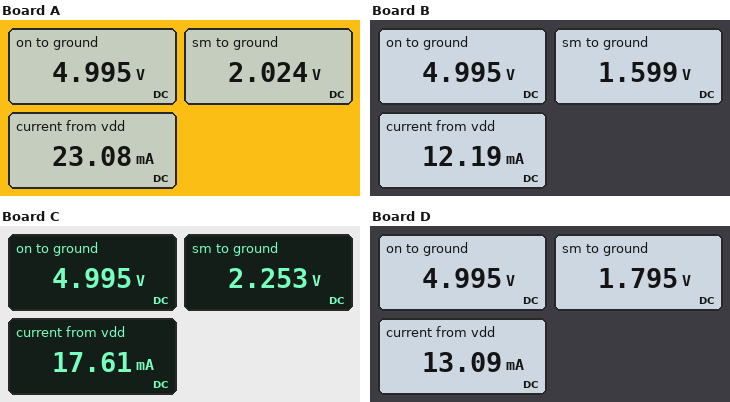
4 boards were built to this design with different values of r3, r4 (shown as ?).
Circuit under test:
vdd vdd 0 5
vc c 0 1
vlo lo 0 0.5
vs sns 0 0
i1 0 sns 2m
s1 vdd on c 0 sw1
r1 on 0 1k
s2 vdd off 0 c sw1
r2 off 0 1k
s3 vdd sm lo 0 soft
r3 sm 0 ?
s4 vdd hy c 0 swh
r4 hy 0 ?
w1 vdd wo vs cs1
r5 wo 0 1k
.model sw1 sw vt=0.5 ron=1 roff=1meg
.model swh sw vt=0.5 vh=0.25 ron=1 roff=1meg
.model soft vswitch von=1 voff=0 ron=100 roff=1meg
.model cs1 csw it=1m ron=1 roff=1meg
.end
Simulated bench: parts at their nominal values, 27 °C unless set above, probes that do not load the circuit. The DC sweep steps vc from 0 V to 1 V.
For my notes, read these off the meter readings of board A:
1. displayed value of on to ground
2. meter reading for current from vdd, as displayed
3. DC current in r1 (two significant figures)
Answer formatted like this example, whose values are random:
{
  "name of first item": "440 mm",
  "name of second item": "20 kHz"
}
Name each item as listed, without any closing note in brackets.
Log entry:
{
  "displayed value of on to ground": "4.995 V",
  "meter reading for current from vdd, as displayed": "23.08 mA",
  "DC current in r1": "5.0 mA"
}
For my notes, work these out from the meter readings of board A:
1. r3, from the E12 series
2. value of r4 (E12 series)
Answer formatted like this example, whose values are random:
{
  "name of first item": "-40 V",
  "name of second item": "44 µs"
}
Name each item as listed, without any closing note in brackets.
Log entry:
{
  "r3, from the E12 series": "6.8 kΩ",
  "value of r4": "390 Ω"
}
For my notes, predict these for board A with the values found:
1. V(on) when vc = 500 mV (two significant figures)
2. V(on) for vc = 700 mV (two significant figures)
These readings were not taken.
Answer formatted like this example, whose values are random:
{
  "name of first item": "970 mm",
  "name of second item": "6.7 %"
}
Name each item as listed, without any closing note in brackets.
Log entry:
{
  "V(on) when vc = 500 mV": "5.0 V",
  "V(on) for vc = 700 mV": "5.0 V"
}
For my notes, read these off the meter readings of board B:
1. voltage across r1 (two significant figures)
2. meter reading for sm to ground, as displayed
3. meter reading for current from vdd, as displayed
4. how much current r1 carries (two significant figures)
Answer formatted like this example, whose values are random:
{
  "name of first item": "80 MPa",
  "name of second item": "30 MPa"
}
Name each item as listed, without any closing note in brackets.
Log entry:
{
  "voltage across r1": "5.0 V",
  "meter reading for sm to ground, as displayed": "1.599 V",
  "meter reading for current from vdd, as displayed": "12.19 mA",
  "how much current r1 carries": "5.0 mA"
}
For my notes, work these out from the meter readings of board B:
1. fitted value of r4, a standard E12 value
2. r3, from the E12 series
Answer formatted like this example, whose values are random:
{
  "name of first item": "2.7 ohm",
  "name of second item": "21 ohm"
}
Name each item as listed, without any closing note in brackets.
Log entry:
{
  "fitted value of r4, a standard E12 value": "2.7 kΩ",
  "r3, from the E12 series": "4.7 kΩ"
}
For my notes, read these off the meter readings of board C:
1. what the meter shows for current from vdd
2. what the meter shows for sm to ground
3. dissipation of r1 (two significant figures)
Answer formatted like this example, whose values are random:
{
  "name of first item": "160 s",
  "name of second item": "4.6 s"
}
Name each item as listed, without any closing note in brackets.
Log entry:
{
  "what the meter shows for current from vdd": "17.61 mA",
  "what the meter shows for sm to ground": "2.253 V",
  "dissipation of r1": "25 mW"
}
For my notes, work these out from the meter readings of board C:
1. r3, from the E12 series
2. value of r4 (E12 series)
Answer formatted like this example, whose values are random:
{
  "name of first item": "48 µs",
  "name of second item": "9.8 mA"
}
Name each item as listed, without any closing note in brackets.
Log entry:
{
  "r3, from the E12 series": "8.2 kΩ",
  "value of r4": "680 Ω"
}
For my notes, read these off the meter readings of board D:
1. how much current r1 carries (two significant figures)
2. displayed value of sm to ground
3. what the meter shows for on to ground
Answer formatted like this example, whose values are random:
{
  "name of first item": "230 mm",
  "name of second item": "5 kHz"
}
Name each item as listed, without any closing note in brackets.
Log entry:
{
  "how much current r1 carries": "5.0 mA",
  "displayed value of sm to ground": "1.795 V",
  "what the meter shows for on to ground": "4.995 V"
}
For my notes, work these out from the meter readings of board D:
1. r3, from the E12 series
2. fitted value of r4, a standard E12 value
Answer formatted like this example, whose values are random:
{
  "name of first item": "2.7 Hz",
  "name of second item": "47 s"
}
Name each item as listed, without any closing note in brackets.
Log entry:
{
  "r3, from the E12 series": "5.6 kΩ",
  "fitted value of r4, a standard E12 value": "1.8 kΩ"
}
